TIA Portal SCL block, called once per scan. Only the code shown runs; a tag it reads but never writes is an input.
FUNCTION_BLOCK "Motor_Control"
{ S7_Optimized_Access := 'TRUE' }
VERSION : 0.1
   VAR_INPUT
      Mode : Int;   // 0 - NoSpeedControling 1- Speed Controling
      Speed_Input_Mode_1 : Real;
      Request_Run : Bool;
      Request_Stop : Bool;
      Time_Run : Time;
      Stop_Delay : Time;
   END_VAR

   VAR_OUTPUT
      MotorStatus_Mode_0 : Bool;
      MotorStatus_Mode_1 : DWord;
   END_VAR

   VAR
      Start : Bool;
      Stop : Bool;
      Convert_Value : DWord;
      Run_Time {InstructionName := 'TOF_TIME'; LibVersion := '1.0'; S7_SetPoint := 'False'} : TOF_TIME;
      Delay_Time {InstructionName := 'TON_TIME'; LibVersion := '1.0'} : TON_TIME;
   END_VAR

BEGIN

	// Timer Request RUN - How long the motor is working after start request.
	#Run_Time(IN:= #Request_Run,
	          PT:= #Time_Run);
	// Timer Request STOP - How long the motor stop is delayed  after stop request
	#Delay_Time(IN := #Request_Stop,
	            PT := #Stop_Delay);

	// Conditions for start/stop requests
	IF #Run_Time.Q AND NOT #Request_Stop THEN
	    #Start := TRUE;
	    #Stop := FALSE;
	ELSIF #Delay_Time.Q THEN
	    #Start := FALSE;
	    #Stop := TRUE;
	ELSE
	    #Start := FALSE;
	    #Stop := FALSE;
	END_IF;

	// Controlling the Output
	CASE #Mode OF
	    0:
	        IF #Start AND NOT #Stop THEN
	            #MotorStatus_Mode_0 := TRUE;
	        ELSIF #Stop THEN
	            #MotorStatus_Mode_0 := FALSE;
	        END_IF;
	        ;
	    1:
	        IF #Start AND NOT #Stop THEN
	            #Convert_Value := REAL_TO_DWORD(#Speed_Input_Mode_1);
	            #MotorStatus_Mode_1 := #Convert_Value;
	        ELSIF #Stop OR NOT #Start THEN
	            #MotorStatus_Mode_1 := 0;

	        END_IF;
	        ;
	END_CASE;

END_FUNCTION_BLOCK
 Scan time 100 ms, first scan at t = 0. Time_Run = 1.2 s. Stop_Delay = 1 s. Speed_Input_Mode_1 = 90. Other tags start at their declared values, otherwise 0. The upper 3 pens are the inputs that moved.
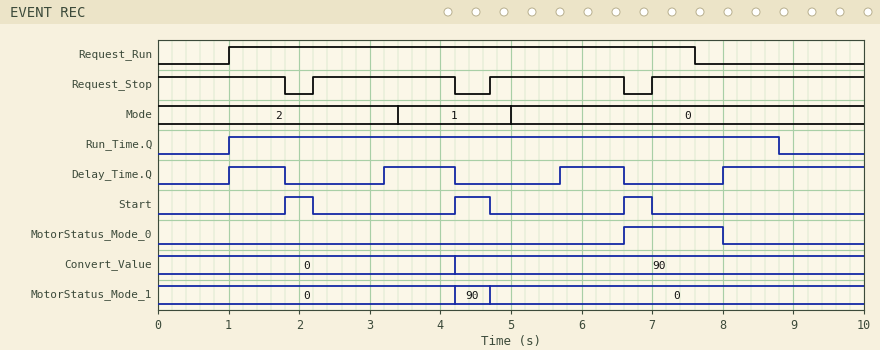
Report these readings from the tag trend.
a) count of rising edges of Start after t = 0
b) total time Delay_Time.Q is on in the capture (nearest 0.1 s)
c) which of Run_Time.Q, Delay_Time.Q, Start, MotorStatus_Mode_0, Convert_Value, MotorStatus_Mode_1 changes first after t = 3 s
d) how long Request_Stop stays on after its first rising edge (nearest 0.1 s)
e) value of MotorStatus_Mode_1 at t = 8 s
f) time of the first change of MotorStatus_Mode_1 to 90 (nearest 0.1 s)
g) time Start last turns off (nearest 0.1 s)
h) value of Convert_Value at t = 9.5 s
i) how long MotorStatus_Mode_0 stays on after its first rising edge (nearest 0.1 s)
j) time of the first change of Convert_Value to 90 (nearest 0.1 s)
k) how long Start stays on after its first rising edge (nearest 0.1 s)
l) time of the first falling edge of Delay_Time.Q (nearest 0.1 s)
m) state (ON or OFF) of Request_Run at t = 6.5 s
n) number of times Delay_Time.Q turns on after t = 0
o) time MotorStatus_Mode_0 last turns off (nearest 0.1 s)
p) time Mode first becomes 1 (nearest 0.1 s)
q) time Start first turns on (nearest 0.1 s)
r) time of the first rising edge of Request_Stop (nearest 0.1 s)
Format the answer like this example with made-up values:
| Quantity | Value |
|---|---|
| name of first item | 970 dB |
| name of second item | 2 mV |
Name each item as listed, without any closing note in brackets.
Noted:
| Quantity | Value |
|---|---|
| count of rising edges of Start after t = 0 | 3 |
| total time Delay_Time.Q is on in the capture | 4.7 s |
| which of Run_Time.Q, Delay_Time.Q, Start, MotorStatus_Mode_0, Convert_Value, MotorStatus_Mode_1 changes first after t = 3 s | Delay_Time.Q |
| how long Request_Stop stays on after its first rising edge | 2.0 s |
| value of MotorStatus_Mode_1 at t = 8 s | 0 |
| time of the first change of MotorStatus_Mode_1 to 90 | 4.2 s |
| time Start last turns off | 7.0 s |
| value of Convert_Value at t = 9.5 s | 90 |
| how long MotorStatus_Mode_0 stays on after its first rising edge | 1.4 s |
| time of the first change of Convert_Value to 90 | 4.2 s |
| how long Start stays on after its first rising edge | 0.4 s |
| time of the first falling edge of Delay_Time.Q | 1.8 s |
| state (ON or OFF) of Request_Run at t = 6.5 s | ON |
| number of times Delay_Time.Q turns on after t = 0 | 4 |
| time MotorStatus_Mode_0 last turns off | 8.0 s |
| time Mode first becomes 1 | 3.4 s |
| time Start first turns on | 1.8 s |
| time of the first rising edge of Request_Stop | 2.2 s |
